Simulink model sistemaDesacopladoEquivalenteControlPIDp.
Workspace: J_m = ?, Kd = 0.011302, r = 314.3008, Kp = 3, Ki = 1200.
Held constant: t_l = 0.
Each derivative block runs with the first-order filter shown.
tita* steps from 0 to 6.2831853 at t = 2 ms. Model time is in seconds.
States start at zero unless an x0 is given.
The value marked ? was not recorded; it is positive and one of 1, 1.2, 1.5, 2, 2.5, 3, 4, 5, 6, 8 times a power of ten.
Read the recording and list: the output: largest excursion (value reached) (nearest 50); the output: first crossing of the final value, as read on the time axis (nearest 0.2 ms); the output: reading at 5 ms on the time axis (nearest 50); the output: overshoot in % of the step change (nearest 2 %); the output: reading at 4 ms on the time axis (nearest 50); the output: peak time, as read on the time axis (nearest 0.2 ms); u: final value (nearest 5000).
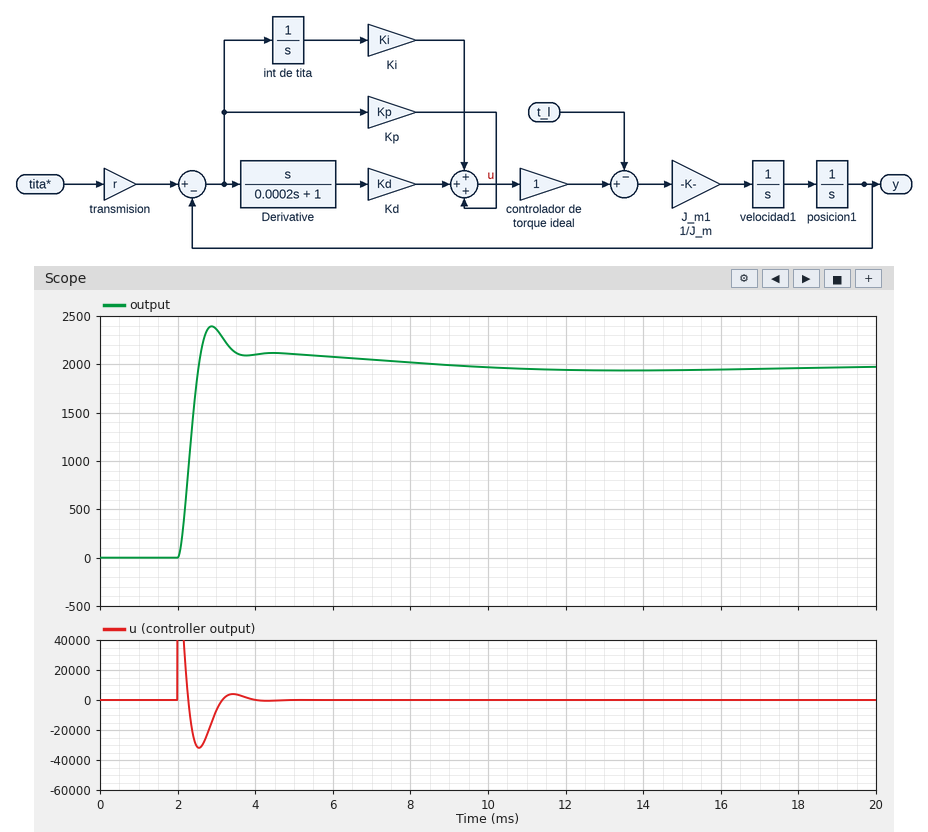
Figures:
2400
2.6 ms
2100
22 %
2100
2.8 ms
0
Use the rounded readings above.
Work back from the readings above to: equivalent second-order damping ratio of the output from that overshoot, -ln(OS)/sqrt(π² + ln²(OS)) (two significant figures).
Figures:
0.43
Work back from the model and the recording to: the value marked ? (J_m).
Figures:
3e-06
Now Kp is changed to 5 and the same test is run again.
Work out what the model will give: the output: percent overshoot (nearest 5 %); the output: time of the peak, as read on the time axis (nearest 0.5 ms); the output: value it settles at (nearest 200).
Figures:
25 %
3.0 ms
2000
